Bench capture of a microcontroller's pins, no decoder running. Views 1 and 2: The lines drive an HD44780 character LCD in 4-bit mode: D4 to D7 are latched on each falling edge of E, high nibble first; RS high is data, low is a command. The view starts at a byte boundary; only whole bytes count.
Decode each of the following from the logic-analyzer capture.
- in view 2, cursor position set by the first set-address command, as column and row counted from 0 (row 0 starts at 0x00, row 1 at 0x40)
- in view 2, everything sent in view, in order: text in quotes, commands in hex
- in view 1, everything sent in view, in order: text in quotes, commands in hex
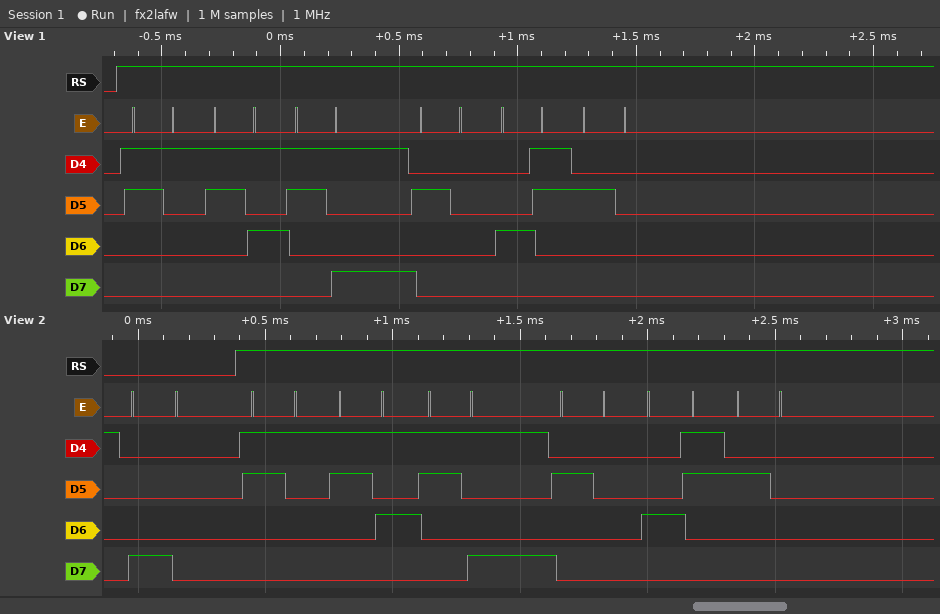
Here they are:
column 0, row 0
0x80 "159 C "
"159 C "
